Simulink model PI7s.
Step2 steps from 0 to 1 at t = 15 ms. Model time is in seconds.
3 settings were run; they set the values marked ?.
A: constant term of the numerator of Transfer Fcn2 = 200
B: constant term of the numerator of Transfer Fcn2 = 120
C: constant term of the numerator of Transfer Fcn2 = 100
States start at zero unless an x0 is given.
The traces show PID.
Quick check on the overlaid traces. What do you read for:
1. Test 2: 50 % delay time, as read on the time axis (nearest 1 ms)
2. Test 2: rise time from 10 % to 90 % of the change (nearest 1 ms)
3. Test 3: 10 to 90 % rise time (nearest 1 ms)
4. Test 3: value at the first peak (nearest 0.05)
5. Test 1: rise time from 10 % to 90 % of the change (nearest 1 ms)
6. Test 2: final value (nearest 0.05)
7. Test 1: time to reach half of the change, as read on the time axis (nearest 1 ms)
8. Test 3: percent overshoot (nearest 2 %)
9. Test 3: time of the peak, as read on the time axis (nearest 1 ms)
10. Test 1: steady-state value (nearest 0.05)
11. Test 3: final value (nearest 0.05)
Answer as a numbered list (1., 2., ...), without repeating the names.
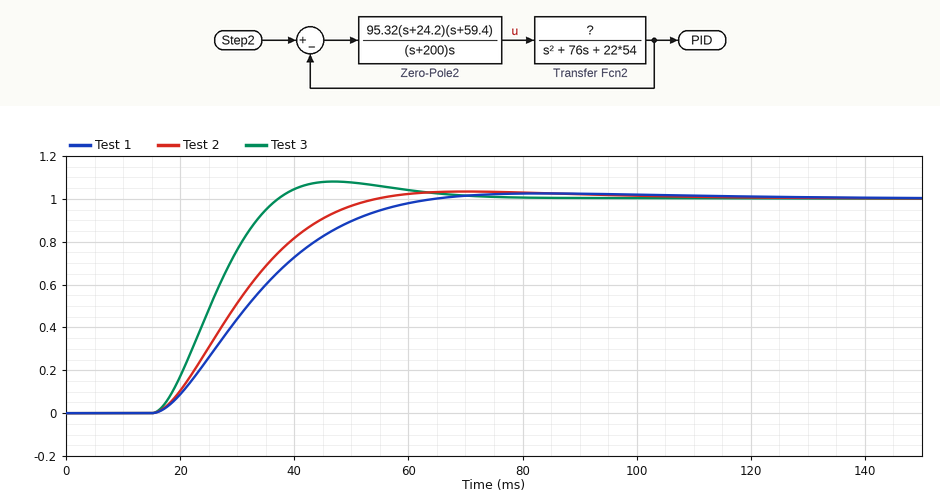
1. 30 ms
2. 25 ms
3. 15 ms
4. 1.10
5. 30 ms
6. 1.00
7. 32 ms
8. 8 %
9. 47 ms
10. 1.00
11. 1.00
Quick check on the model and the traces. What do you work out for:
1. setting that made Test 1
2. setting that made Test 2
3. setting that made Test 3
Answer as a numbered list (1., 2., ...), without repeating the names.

1. C
2. B
3. A
